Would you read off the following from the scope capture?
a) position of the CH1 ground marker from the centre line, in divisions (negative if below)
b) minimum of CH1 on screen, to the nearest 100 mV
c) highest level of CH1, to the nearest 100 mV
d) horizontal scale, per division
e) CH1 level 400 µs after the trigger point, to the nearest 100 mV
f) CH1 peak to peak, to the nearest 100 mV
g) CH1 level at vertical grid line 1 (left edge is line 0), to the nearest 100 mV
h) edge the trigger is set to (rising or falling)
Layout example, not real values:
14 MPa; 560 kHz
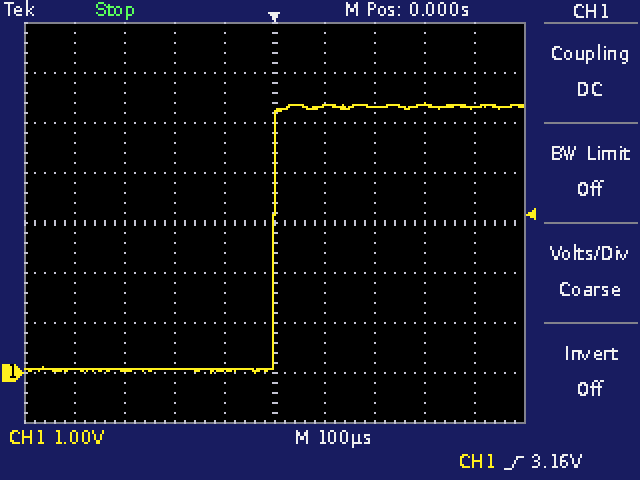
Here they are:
-3.0 div; 0.0 V; 5.4 V; 100 µs; 5.3 V; 5.4 V; 100 mV; rising
